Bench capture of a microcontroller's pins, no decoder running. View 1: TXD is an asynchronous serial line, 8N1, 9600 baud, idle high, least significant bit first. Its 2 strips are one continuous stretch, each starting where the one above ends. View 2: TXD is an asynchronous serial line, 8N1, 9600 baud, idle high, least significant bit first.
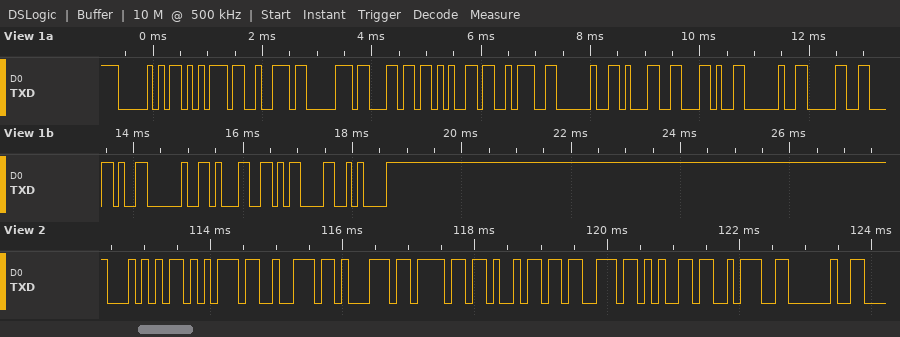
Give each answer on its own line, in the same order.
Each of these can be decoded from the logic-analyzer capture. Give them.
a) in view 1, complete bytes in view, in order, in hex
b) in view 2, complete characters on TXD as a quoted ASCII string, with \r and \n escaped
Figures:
50 75 72 70 6C 65 3A 20 31 2C 20 30 2C 20 31 0D 0A
"Turqoise: "
